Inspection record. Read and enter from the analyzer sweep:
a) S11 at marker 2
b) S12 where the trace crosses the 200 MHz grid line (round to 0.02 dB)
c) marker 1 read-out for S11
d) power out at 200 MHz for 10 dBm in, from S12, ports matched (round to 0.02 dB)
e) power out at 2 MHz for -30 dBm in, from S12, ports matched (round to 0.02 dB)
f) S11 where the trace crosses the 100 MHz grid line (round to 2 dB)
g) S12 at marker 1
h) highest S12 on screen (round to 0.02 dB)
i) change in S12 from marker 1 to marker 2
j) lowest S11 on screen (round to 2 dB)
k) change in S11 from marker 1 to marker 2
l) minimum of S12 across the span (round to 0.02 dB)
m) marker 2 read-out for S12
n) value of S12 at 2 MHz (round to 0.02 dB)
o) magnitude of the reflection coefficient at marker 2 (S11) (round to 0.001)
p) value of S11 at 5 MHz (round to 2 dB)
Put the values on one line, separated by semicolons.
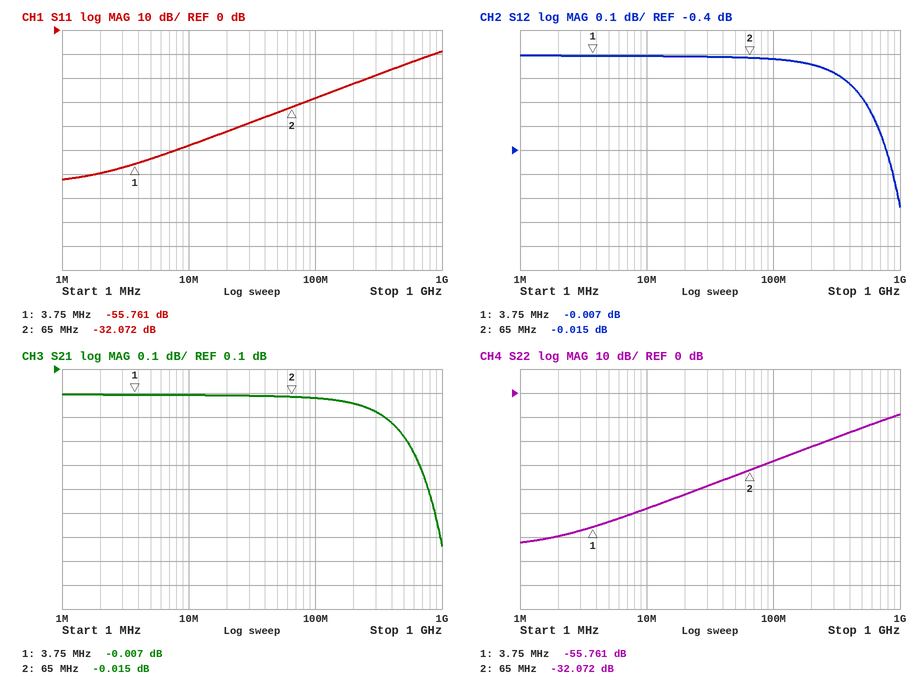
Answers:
-32.072 dB; -0.04 dB; -55.761 dB; 9.96 dBm; -30.00 dBm; -28 dB; -0.007 dB; 0.00 dB; -0.008 dB; -62 dB; 23.689 dB; -0.64 dB; -0.015 dB; 0.00 dB; 0.025; -54 dB
